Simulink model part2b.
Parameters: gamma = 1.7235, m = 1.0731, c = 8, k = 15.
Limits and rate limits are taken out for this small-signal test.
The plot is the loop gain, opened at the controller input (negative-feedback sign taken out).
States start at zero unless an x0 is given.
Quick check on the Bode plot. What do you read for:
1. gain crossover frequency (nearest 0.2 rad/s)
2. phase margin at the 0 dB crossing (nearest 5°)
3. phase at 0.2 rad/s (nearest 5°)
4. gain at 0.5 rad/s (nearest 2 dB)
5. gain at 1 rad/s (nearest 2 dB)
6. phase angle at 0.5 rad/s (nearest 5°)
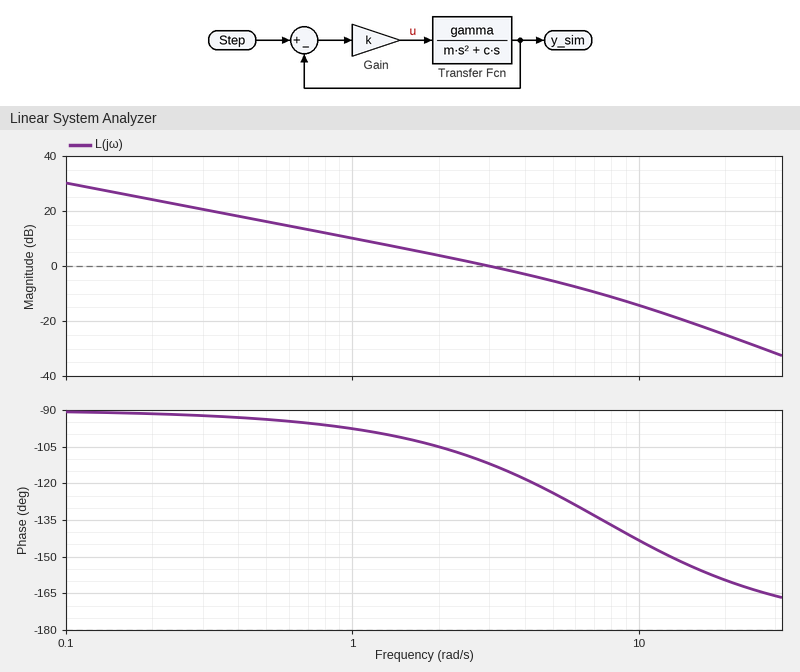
3.0 rad/s
70°
-90°
16 dB
10 dB
-95°
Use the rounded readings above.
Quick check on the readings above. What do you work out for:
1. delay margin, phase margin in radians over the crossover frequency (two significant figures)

0.41 s
